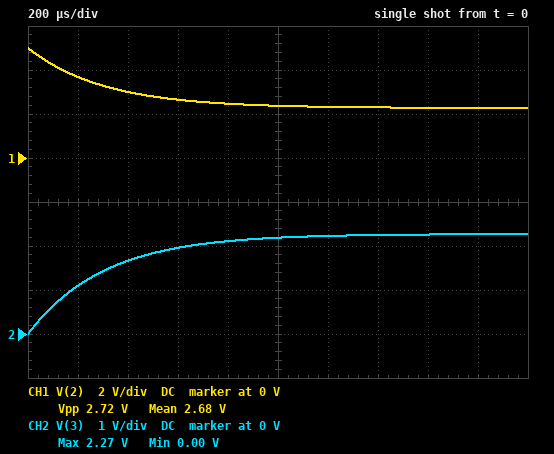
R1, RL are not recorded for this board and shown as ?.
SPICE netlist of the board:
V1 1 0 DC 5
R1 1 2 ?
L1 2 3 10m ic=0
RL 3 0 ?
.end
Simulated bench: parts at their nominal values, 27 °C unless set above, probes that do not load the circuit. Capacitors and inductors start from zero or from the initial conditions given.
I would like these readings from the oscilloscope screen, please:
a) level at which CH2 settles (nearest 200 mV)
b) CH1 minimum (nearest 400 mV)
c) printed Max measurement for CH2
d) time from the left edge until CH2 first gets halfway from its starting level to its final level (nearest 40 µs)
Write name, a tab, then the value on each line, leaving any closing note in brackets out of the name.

level at which CH2 settles	2.2 V
CH1 minimum	2.4 V
printed Max measurement for CH2	2.27 V
time from the left edge until CH2 first gets halfway from its starting level to its final level	200 µs
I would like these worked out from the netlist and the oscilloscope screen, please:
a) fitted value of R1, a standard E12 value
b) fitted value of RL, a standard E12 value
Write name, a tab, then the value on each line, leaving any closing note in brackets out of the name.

fitted value of R1, a standard E12 value	18 Ω
fitted value of RL, a standard E12 value	15 Ω
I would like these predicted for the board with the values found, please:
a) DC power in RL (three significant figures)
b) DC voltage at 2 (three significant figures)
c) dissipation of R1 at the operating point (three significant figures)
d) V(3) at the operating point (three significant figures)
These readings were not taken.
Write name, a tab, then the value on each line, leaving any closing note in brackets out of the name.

DC power in RL	344 mW
DC voltage at 2	2.27 V
dissipation of R1 at the operating point	413 mW
V(3) at the operating point	2.27 V
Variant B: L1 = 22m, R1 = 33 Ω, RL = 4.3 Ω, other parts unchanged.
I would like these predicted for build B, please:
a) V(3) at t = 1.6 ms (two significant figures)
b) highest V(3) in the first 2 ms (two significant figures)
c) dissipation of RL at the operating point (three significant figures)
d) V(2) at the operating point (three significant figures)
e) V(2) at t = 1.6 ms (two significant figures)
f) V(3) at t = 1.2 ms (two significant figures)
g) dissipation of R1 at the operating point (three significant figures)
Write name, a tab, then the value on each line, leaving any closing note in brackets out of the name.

V(3) at t = 1.6 ms	540 mV
highest V(3) in the first 2 ms	560 mV
dissipation of RL at the operating point	77.3 mW
V(2) at the operating point	576 mV
V(2) at t = 1.6 ms	870 mV
V(3) at t = 1.2 ms	500 mV
dissipation of R1 at the operating point	593 mW
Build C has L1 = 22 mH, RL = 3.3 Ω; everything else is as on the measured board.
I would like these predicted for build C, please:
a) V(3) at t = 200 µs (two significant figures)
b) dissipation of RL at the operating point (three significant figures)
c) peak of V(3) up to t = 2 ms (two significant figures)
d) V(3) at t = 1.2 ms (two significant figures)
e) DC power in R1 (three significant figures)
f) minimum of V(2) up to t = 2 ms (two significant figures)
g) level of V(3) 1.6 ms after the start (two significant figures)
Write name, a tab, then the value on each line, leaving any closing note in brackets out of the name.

V(3) at t = 200 µs	140 mV
dissipation of RL at the operating point	182 mW
peak of V(3) up to t = 2 ms	660 mV
V(3) at t = 1.2 ms	530 mV
DC power in R1	992 mW
minimum of V(2) up to t = 2 ms	1.4 V
level of V(3) 1.6 ms after the start	610 mV
